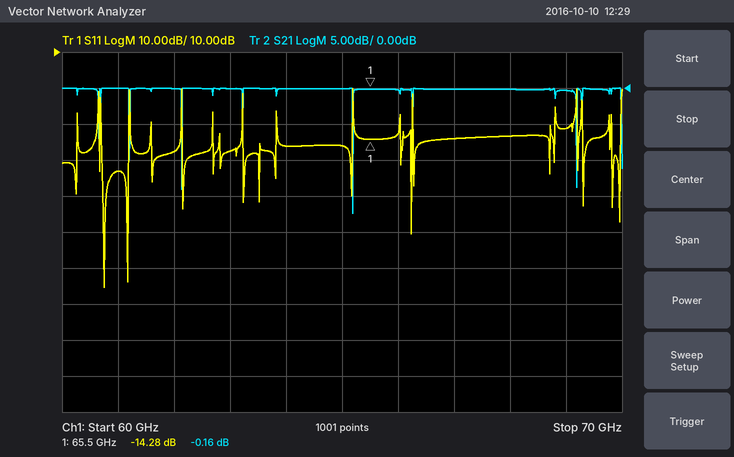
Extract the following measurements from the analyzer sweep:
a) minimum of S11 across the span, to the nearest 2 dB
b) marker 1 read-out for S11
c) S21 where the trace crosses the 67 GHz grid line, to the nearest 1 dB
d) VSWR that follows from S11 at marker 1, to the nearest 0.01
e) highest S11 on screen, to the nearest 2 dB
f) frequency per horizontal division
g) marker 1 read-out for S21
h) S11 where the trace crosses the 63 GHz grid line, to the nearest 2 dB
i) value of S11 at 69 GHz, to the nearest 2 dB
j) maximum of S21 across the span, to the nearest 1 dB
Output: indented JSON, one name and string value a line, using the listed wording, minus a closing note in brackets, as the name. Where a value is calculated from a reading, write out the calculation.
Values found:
{
  "minimum of S11 across the span, to the nearest 2 dB": "-56 dB",
  "marker 1 read-out for S11": "-14.28 dB",
  "S21 where the trace crosses the 67 GHz grid line, to the nearest 1 dB": "0 dB",
  "VSWR that follows from S11 at marker 1, to the nearest 0.01": "(1 + 0.1932)/(1 − 0.1932) ≈ 1.48",
  "highest S11 on screen, to the nearest 2 dB": "0 dB",
  "frequency per horizontal division": "1 GHz",
  "marker 1 read-out for S21": "-0.16 dB",
  "S11 where the trace crosses the 63 GHz grid line, to the nearest 2 dB": "-18 dB",
  "value of S11 at 69 GHz, to the nearest 2 dB": "-12 dB",
  "maximum of S21 across the span, to the nearest 1 dB": "0 dB"
}
